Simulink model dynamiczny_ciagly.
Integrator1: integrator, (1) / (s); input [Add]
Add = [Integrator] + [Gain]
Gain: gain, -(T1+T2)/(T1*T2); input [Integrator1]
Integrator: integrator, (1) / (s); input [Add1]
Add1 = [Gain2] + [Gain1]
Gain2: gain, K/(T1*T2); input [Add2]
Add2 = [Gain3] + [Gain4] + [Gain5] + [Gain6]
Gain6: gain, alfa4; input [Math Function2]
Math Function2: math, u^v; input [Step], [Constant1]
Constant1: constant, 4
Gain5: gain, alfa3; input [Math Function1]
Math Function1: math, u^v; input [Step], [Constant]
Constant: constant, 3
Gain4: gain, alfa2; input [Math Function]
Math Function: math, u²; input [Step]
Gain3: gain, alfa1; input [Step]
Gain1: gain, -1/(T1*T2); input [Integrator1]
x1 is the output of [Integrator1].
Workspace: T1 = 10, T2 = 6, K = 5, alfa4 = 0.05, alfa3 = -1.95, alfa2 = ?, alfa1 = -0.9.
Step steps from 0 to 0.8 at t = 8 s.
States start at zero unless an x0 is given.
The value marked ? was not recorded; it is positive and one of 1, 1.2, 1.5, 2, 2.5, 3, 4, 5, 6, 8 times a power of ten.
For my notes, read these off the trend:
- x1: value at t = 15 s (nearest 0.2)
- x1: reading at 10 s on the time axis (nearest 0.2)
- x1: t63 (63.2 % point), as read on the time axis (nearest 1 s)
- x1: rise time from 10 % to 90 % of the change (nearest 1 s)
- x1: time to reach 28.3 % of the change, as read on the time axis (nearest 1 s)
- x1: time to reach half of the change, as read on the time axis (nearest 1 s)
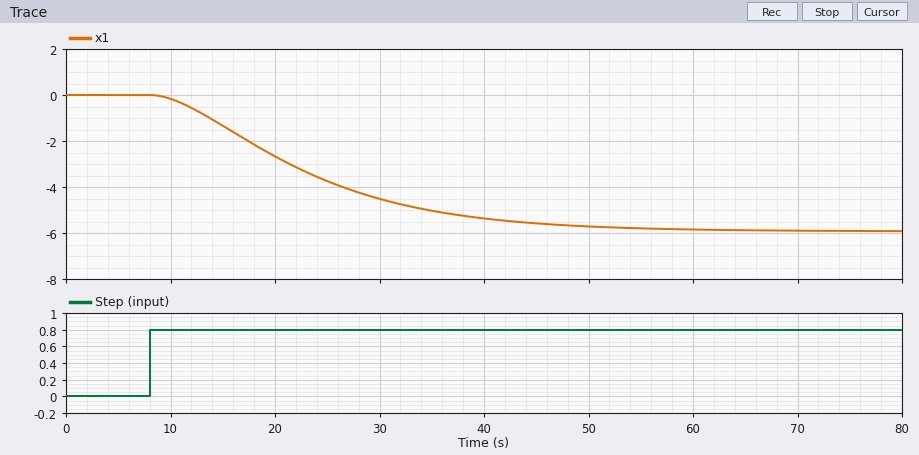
-1.4
-0.2
25 s
27 s
16 s
21 s
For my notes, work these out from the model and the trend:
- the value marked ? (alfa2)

0.8
